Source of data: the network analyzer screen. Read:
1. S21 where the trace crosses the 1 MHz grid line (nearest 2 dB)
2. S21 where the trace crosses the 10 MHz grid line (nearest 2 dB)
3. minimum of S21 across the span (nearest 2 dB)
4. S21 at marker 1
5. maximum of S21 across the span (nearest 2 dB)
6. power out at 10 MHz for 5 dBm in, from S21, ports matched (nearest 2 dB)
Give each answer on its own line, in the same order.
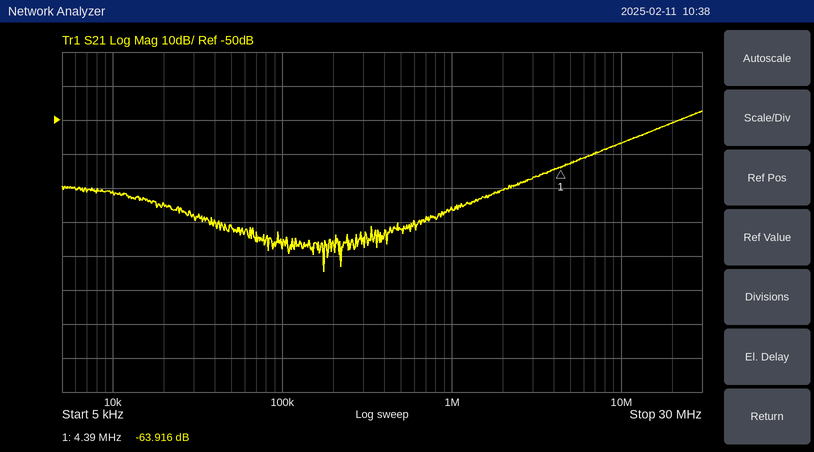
-76 dB
-56 dB
-94 dB
-63.916 dB
-48 dB
-52 dBm
